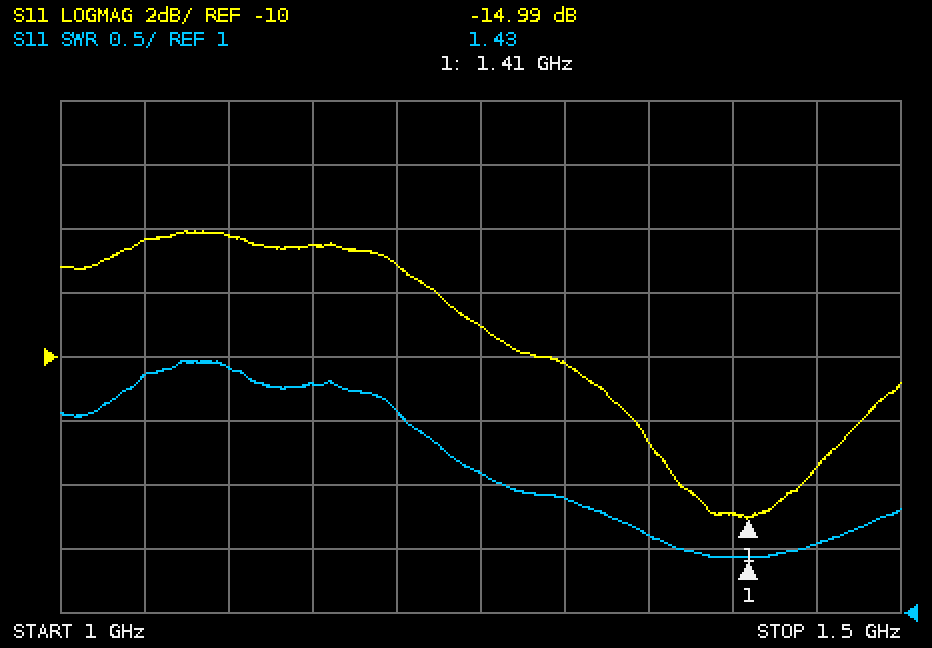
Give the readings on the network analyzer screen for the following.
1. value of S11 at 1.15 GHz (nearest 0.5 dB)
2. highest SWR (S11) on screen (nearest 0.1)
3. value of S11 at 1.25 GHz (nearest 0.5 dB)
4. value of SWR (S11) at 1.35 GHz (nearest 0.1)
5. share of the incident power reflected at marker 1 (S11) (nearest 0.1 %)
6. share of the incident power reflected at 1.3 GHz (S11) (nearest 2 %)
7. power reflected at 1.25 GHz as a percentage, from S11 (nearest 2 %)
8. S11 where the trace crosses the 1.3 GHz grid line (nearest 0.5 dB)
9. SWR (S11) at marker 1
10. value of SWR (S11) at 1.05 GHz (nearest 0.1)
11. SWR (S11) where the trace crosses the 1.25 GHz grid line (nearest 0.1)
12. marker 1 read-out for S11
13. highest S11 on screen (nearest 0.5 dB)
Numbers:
-6.5 dB
3.0
-9.0 dB
1.6
3.2 %
10 %
12 %
-10.0 dB
1.43
2.9
2.1
-14.99 dB
-6.0 dB
